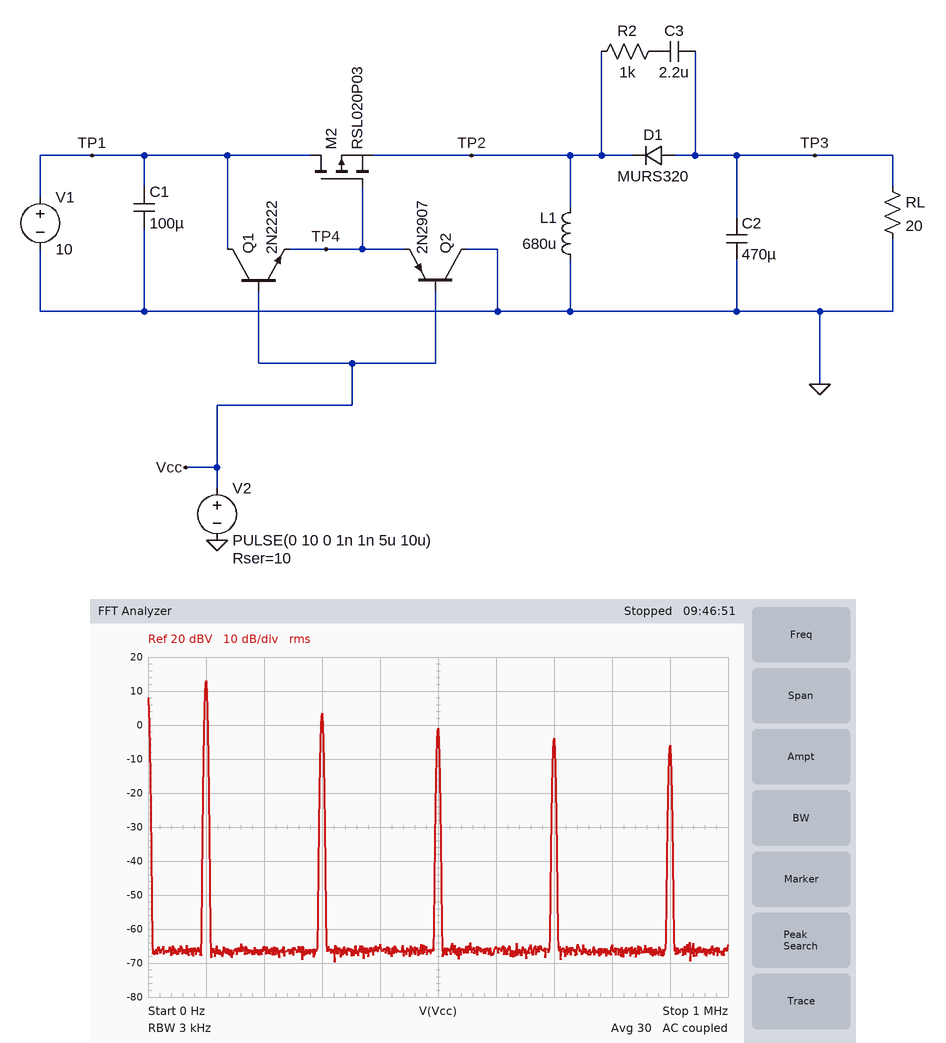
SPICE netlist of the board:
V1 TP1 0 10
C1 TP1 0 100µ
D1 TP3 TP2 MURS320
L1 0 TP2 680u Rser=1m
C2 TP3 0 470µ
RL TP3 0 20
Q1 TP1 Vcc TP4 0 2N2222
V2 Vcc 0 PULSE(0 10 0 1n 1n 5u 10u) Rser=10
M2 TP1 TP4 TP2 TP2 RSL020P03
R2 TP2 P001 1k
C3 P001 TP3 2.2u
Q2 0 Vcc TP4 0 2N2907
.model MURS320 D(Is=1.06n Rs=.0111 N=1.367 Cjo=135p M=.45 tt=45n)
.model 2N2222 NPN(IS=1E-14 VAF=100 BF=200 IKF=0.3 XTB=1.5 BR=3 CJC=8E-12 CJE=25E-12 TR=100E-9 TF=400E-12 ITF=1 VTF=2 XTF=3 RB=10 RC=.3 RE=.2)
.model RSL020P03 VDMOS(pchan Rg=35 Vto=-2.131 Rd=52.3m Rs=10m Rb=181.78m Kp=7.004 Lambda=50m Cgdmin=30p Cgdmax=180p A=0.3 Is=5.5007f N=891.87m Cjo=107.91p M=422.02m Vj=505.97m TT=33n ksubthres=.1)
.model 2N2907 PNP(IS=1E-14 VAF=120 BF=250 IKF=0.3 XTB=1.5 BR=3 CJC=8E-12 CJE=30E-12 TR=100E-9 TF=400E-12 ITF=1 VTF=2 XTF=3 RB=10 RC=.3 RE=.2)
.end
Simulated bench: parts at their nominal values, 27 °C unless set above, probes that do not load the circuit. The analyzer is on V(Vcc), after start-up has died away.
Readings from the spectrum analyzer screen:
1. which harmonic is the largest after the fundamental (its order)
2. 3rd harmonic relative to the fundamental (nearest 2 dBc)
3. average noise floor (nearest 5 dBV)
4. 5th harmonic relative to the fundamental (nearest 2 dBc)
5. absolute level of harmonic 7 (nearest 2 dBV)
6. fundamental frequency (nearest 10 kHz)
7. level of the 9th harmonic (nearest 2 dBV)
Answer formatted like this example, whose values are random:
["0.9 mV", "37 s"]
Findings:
["3", "-10 dBc", "-65 dBV", "-14 dBc", "-4 dBV", "100 kHz", "-6 dBV"]
